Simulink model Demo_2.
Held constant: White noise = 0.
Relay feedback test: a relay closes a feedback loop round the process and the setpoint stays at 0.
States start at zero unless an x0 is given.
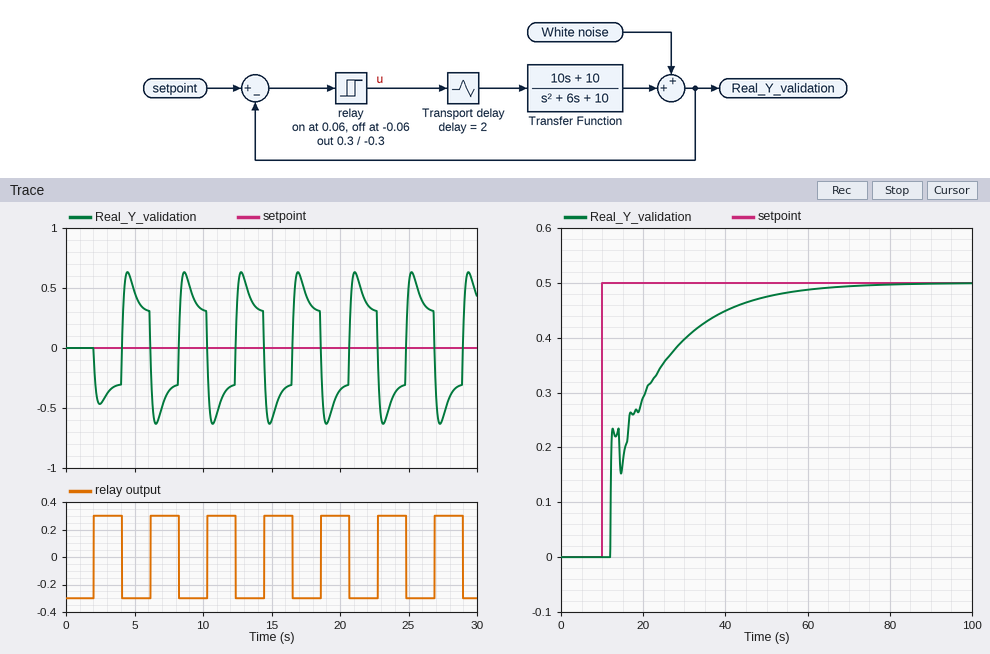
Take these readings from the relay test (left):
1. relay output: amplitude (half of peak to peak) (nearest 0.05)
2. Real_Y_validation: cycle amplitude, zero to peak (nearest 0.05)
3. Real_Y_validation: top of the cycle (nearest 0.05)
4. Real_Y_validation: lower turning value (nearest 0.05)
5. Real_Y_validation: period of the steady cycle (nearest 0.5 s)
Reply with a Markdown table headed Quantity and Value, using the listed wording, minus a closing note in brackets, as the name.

| Quantity | Value |
|---|---|
| relay output: amplitude (half of peak to peak) | 0.30 |
| Real_Y_validation: cycle amplitude, zero to peak | 0.65 |
| Real_Y_validation: top of the cycle | 0.65 |
| Real_Y_validation: lower turning value | -0.65 |
| Real_Y_validation: period of the steady cycle | 4.0 s |
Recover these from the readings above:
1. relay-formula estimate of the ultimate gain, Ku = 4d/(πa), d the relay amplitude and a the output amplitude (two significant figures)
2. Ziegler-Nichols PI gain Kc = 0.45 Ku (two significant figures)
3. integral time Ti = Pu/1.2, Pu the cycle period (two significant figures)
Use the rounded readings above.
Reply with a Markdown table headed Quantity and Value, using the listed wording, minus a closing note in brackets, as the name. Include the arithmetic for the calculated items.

| Quantity | Value |
|---|---|
| relay-formula estimate of the ultimate gain, Ku = 4d/(πa), d the relay amplitude and a the output amplitude | 4 × 0.3 / (π × 0.65) = 0.59 |
| Ziegler-Nichols PI gain Kc = 0.45 Ku | 0.45 × 0.59 = 0.27 |
| integral time Ti = Pu/1.2, Pu the cycle period | 4 / 1.2 = 3.3 s |
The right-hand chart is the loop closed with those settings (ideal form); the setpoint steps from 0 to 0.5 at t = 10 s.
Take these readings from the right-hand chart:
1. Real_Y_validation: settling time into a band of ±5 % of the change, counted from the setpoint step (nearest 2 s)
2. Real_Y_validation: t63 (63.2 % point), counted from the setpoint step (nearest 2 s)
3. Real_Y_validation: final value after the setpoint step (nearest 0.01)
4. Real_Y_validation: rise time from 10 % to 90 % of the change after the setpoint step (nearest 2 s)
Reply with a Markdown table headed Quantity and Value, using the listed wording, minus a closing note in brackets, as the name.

| Quantity | Value |
|---|---|
| Real_Y_validation: settling time into a band of ±5 % of the change, counted from the setpoint step | 40 s |
| Real_Y_validation: t63 (63.2 % point), counted from the setpoint step | 12 s |
| Real_Y_validation: final value after the setpoint step | 0.50 |
| Real_Y_validation: rise time from 10 % to 90 % of the change after the setpoint step | 28 s |
